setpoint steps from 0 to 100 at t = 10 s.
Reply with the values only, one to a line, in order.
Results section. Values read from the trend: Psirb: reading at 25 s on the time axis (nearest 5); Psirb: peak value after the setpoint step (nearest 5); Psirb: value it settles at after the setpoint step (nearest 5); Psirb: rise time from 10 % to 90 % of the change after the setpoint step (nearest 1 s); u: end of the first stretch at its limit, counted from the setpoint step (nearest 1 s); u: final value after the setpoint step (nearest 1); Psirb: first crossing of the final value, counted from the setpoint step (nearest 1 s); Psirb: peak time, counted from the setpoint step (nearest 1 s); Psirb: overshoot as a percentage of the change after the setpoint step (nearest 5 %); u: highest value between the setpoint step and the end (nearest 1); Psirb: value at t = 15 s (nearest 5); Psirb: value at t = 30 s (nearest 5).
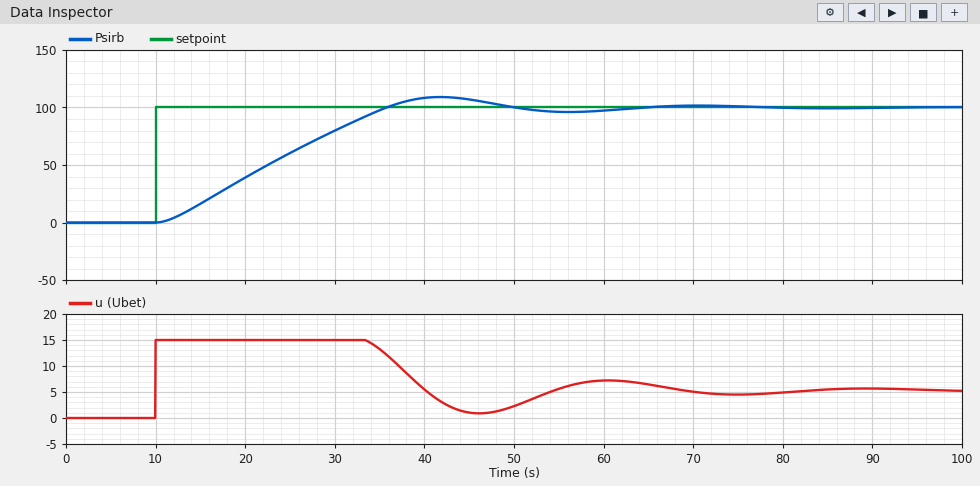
60
110
100
19 s
24 s
5
26 s
32 s
10 %
15
15
80
